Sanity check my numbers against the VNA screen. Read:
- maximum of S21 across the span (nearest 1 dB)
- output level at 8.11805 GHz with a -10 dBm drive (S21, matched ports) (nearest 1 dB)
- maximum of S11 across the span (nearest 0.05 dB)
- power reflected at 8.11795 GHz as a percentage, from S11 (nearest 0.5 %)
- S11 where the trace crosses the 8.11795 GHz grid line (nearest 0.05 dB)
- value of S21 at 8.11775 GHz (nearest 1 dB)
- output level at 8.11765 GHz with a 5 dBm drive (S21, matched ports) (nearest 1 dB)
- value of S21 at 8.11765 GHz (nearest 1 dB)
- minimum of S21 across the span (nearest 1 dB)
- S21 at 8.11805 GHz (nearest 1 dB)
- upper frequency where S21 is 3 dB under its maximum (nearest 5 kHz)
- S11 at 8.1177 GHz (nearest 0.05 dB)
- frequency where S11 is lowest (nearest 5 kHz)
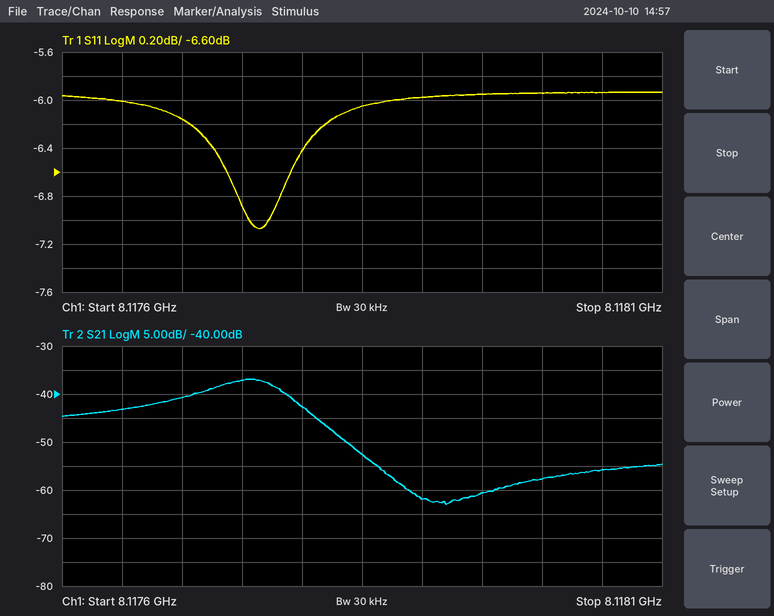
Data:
-37 dB
-66 dBm
-5.95 dB
25.5 %
-5.95 dB
-37 dB
-38 dBm
-43 dB
-63 dB
-56 dB
8.117785 GHz
-6.15 dB
8.117765 GHz
